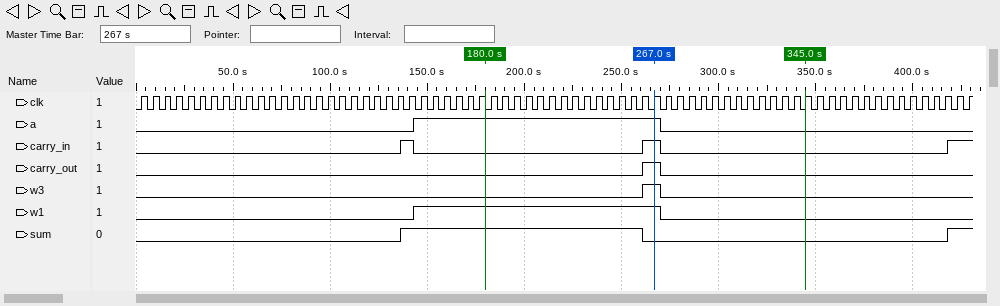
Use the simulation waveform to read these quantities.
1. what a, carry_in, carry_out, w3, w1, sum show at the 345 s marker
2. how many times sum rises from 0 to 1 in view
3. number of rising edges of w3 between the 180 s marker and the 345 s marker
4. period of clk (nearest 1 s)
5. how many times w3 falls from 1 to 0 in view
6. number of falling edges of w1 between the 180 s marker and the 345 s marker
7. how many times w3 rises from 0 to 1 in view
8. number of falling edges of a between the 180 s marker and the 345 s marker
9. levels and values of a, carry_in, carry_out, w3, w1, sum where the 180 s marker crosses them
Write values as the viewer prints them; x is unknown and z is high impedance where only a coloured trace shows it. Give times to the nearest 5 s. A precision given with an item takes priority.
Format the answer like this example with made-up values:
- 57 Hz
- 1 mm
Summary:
- a=0, carry_in=0, carry_out=0, w3=0, w1=0, sum=0
- 2
- 1
- 6 s
- 1
- 1
- 1
- 1
- a=1, carry_in=0, carry_out=0, w3=0, w1=1, sum=1
